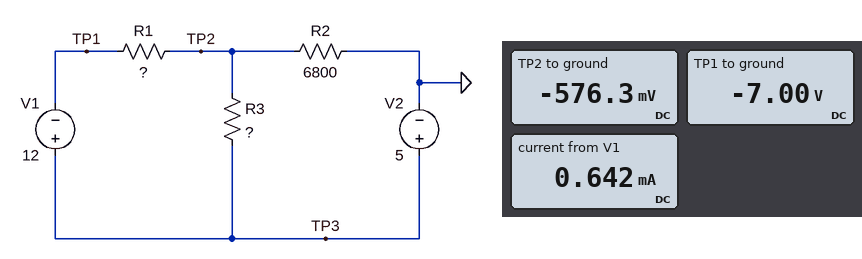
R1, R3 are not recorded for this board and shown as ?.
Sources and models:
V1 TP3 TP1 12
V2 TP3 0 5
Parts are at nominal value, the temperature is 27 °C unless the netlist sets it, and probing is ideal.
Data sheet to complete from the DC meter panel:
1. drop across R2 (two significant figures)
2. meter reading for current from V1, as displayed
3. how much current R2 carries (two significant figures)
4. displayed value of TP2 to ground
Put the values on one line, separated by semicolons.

580 mV; 0.642 mA; 85 µA; -576.3 mV
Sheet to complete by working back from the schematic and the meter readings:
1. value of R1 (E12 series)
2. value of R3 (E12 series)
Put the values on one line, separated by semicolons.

10 kΩ; 10 kΩ
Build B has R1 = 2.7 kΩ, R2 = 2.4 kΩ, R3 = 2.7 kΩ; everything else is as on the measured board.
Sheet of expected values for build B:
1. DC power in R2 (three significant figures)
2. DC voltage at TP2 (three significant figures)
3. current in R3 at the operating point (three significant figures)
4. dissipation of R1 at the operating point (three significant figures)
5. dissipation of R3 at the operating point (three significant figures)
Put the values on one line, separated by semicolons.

171 µW; -640 mV; 2.09 mA; 15.0 mW; 11.8 mW
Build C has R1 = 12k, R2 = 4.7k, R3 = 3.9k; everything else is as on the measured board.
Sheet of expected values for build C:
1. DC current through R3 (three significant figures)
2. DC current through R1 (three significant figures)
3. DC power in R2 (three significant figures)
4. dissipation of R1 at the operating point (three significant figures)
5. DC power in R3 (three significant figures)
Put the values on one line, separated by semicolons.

958 µA; 689 µA; 340 µW; 5.69 mW; 3.58 mW
